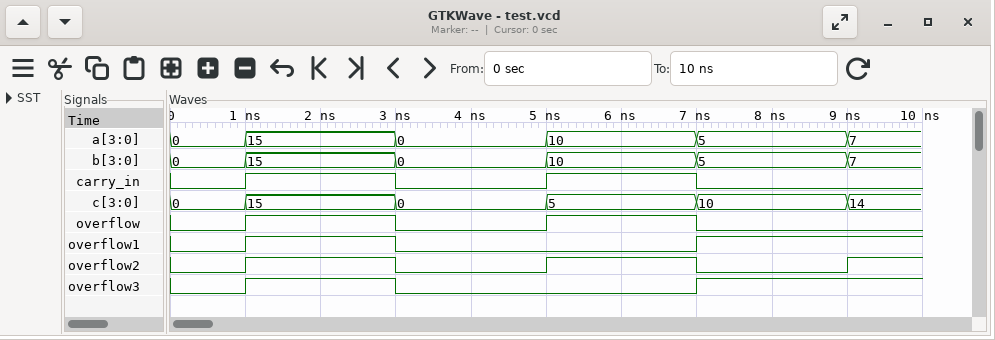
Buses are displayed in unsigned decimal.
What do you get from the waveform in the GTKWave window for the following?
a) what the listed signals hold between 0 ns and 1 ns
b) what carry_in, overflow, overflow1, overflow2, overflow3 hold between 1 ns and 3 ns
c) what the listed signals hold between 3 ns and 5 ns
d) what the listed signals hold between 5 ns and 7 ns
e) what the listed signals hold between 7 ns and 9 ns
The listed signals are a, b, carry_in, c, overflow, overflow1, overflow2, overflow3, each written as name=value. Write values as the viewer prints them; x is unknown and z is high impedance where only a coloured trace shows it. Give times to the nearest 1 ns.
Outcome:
a=0, b=0, carry_in=0, c=0, overflow=0, overflow1=0, overflow2=0, overflow3=0
carry_in=1, overflow=1, overflow1=1, overflow2=1, overflow3=1
a=0, b=0, carry_in=0, c=0, overflow=0, overflow1=0, overflow2=0, overflow3=0
a=10, b=10, carry_in=1, c=5, overflow=1, overflow1=0, overflow2=1, overflow3=0
a=5, b=5, carry_in=0, c=10, overflow=0, overflow1=1, overflow2=0, overflow3=1
